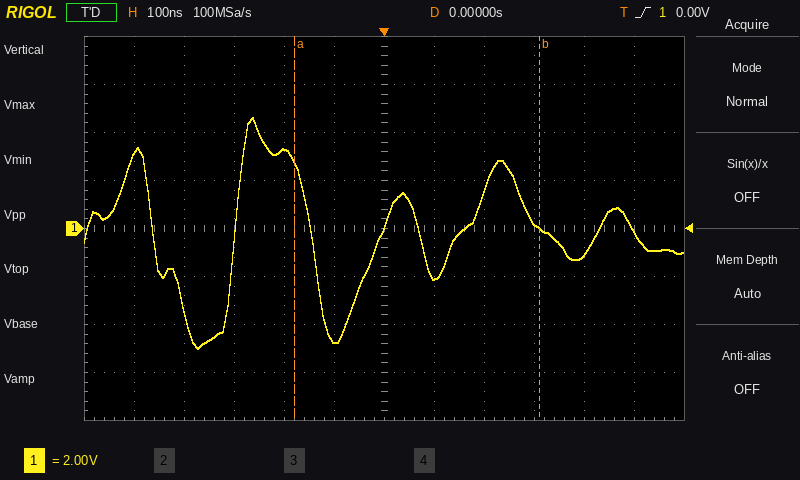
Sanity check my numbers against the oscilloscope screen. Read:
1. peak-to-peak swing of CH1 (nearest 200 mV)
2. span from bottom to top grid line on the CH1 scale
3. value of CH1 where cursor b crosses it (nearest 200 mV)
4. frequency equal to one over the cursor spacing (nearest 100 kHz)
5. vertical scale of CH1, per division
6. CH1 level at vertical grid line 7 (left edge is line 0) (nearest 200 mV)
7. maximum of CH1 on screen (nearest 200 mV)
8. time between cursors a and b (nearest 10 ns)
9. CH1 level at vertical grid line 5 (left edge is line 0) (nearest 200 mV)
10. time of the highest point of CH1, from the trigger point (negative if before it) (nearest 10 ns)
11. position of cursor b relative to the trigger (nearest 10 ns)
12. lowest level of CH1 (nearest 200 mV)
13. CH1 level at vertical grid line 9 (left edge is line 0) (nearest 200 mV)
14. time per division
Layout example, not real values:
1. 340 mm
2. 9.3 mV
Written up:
1. 9.6 V
2. 16 V
3. 0.0 V
4. 2.0 MHz
5. 2 V
6. -2.0 V
7. 4.6 V
8. 490 ns
9. -4.6 V
10. -260 ns
11. +310 ns
12. -5.0 V
13. 200 mV
14. 100 ns
